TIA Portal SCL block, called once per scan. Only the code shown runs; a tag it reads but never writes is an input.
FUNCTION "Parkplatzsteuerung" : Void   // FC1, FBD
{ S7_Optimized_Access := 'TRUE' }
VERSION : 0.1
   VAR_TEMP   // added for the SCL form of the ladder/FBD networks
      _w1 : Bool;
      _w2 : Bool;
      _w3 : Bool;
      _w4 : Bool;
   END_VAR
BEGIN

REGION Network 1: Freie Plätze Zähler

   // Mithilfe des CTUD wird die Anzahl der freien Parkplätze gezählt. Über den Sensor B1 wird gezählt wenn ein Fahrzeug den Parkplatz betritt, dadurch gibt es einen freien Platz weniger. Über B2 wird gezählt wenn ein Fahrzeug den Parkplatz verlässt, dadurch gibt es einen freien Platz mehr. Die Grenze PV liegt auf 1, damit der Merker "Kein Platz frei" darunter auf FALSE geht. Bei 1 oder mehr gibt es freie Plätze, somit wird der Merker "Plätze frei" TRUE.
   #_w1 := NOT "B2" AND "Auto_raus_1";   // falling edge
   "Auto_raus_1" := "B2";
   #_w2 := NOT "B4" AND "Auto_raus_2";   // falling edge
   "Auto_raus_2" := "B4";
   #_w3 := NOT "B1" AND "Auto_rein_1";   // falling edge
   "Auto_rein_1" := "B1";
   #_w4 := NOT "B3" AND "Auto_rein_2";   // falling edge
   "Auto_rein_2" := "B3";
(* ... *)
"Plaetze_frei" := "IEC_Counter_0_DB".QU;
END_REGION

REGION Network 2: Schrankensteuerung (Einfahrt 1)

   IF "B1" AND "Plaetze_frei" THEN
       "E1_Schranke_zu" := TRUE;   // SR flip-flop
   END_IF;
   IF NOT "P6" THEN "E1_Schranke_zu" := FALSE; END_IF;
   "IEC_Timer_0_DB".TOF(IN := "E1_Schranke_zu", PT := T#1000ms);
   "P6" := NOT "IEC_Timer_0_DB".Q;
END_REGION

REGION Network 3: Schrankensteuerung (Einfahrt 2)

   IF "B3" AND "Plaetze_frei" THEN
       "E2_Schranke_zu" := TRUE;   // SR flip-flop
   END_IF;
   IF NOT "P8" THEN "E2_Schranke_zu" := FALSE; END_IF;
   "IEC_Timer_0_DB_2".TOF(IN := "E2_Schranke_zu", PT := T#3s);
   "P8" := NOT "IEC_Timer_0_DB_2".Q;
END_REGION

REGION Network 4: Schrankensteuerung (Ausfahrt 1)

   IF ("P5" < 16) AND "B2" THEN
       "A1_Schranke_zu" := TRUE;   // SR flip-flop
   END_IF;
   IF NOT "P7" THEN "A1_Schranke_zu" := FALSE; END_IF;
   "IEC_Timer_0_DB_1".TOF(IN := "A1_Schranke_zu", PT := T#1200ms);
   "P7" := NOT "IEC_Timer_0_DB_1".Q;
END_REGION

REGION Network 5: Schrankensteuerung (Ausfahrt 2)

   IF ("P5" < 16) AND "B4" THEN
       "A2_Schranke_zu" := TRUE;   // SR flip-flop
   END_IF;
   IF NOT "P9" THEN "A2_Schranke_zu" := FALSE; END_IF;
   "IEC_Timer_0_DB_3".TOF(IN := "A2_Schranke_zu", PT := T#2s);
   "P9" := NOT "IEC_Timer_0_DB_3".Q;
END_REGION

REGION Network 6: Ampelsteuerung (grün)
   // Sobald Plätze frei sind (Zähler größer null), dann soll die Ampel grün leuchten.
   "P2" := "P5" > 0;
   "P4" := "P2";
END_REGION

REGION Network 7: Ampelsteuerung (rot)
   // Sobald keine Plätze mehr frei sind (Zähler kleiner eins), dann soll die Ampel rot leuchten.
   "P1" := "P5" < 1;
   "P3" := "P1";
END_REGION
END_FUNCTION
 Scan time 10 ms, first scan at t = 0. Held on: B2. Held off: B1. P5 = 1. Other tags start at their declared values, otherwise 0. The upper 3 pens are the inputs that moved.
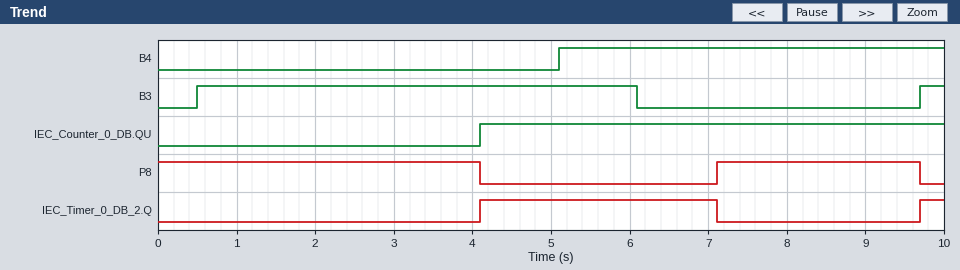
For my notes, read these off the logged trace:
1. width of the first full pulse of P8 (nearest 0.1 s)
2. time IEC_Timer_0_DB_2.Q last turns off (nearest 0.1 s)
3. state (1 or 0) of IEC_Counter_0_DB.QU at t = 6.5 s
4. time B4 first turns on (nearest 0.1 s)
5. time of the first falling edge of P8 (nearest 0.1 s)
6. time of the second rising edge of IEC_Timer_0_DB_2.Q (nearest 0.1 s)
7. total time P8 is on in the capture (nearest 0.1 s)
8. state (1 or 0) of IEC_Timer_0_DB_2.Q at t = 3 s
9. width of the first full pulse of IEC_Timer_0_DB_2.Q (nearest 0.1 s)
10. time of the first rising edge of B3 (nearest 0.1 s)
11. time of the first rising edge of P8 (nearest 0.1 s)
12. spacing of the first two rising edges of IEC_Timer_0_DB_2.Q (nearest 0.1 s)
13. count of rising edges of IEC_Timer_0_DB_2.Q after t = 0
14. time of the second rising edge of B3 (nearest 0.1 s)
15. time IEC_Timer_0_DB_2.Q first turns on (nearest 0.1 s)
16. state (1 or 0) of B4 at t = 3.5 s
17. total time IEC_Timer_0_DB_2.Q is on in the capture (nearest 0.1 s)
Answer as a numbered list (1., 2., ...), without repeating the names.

1. 2.6 s
2. 7.1 s
3. 1
4. 5.1 s
5. 4.1 s
6. 9.7 s
7. 6.7 s
8. 0
9. 3.0 s
10. 0.5 s
11. 7.1 s
12. 5.6 s
13. 2
14. 9.7 s
15. 4.1 s
16. 0
17. 3.3 s
